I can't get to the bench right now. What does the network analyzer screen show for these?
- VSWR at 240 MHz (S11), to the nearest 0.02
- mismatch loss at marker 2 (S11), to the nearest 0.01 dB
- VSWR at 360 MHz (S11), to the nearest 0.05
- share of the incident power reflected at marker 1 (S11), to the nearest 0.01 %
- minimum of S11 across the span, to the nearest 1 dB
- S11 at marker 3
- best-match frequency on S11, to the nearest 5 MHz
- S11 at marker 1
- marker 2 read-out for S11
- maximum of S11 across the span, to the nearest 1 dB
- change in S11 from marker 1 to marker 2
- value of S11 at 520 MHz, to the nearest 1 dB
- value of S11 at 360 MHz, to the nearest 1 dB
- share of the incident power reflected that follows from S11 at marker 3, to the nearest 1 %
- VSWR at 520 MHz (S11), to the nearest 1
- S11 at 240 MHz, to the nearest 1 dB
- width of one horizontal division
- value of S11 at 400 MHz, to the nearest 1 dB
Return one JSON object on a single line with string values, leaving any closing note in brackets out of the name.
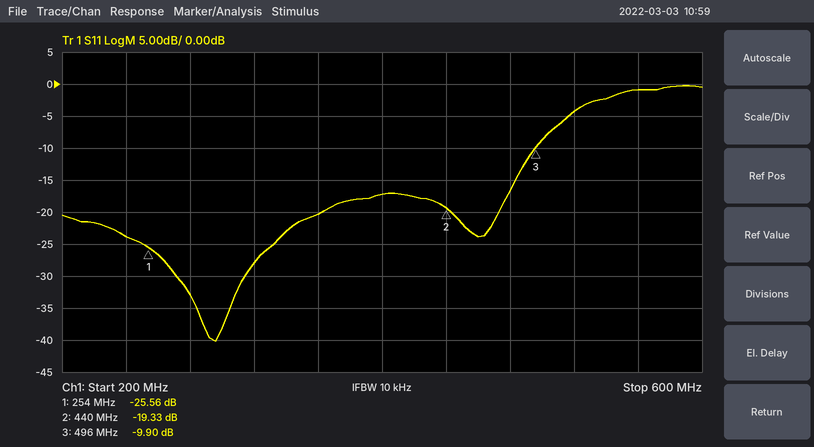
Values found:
{"VSWR at 240 MHz (S11), to the nearest 0.02": "1.14", "mismatch loss at marker 2 (S11), to the nearest 0.01 dB": "0.05 dB", "VSWR at 360 MHz (S11), to the nearest 0.05": "1.20", "share of the incident power reflected at marker 1 (S11), to the nearest 0.01 %": "0.28 %", "minimum of S11 across the span, to the nearest 1 dB": "-40 dB", "S11 at marker 3": "-9.90 dB", "best-match frequency on S11, to the nearest 5 MHz": "295 MHz", "S11 at marker 1": "-25.56 dB", "marker 2 read-out for S11": "-19.33 dB", "maximum of S11 across the span, to the nearest 1 dB": "0 dB", "change in S11 from marker 1 to marker 2": "6.23 dB", "value of S11 at 520 MHz, to the nearest 1 dB": "-4 dB", "value of S11 at 360 MHz, to the nearest 1 dB": "-20 dB", "share of the incident power reflected that follows from S11 at marker 3, to the nearest 1 %": "10 %", "VSWR at 520 MHz (S11), to the nearest 1": "4", "S11 at 240 MHz, to the nearest 1 dB": "-24 dB", "width of one horizontal division": "40 MHz", "value of S11 at 400 MHz, to the nearest 1 dB": "-17 dB"}
